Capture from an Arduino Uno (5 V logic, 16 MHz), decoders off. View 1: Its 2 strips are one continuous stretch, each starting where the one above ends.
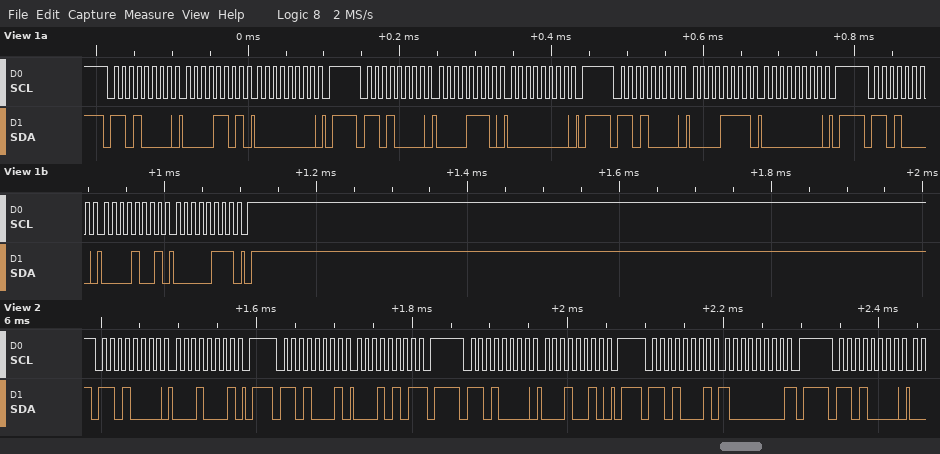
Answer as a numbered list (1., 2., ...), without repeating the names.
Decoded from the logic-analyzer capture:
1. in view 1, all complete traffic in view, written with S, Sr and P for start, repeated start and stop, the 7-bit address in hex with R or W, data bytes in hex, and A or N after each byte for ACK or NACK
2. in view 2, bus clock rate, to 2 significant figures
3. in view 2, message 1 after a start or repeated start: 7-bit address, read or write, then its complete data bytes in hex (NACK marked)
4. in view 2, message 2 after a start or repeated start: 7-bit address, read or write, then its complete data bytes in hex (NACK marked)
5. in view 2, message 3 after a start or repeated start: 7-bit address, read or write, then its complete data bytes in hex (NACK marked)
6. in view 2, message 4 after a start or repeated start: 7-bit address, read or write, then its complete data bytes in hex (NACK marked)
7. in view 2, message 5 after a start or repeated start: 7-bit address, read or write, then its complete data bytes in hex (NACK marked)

1. S 68W A 0D A 00 A P S 68W A 0E A 00 A P S 68W A 0F A 00 A P S 68W A 09 A 07 A P
2. 100 kHz
3. 0x68 write: 11
4. 0x68 read: 15 NACK
5. 0x68 write: 12
6. 0x68 read: 80 NACK
7. 0x68 write
